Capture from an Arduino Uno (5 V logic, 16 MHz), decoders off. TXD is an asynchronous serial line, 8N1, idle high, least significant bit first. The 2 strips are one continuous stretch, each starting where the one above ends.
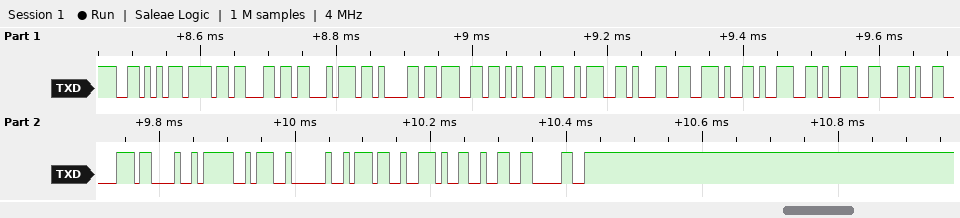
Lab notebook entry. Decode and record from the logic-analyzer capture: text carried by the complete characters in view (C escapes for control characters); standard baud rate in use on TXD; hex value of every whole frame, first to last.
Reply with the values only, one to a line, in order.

"Voltage:1.99,pH: 7.20"
115200 baud
56 6F 6C 74 61 67 65 3A 31 2E 39 39 2C 70 48 3A 20 37 2E 32 30
